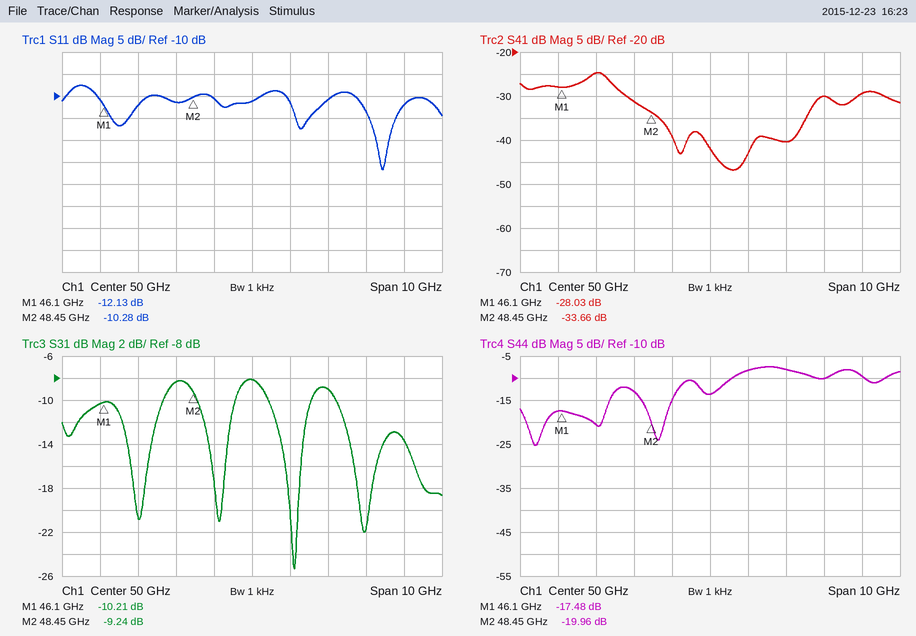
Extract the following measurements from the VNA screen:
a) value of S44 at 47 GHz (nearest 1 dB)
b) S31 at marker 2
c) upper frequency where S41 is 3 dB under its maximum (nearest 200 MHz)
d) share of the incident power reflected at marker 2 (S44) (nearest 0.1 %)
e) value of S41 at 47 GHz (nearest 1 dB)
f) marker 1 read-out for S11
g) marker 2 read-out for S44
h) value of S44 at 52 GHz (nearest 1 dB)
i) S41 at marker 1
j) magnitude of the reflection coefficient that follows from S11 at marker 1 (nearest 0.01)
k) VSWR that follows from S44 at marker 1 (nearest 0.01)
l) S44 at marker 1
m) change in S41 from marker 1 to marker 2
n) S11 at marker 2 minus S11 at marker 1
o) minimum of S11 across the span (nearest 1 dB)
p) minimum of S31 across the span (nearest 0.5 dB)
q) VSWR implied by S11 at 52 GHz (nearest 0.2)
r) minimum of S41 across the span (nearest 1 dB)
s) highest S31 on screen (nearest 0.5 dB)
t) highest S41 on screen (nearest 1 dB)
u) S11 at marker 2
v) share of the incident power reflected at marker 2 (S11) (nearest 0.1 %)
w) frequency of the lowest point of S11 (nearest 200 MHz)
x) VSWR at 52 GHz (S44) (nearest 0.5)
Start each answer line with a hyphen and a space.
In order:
- -21 dB
- -9.24 dB
- 47.4 GHz
- 1.0 %
- -25 dB
- -12.13 dB
- -19.96 dB
- -8 dB
- -28.03 dB
- 0.25
- 1.31
- -17.48 dB
- -5.63 dB
- 1.85 dB
- -27 dB
- -25.5 dB
- 1.8
- -47 dB
- -8.0 dB
- -25 dB
- -10.28 dB
- 9.4 %
- 53.4 GHz
- 2.5
